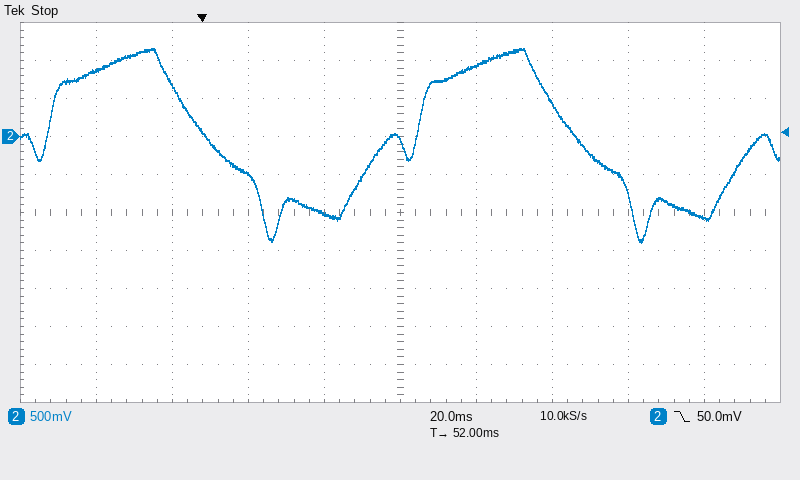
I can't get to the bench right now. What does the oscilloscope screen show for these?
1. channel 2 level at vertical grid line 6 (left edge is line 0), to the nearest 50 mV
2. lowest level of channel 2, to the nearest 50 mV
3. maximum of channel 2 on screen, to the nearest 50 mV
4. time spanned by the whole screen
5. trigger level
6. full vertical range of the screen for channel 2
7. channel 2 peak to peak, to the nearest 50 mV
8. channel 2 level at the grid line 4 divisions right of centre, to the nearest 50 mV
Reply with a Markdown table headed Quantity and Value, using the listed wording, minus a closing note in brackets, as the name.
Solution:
| Quantity | Value |
|---|---|
| channel 2 level at vertical grid line 6 (left edge is line 0), to the nearest 50 mV | 950 mV |
| lowest level of channel 2, to the nearest 50 mV | -1.40 V |
| maximum of channel 2 on screen, to the nearest 50 mV | 1.15 V |
| time spanned by the whole screen | 200 ms |
| trigger level | 50.0 mV |
| full vertical range of the screen for channel 2 | 5 V |
| channel 2 peak to peak, to the nearest 50 mV | 2.55 V |
| channel 2 level at the grid line 4 divisions right of centre, to the nearest 50 mV | -1.05 V |
